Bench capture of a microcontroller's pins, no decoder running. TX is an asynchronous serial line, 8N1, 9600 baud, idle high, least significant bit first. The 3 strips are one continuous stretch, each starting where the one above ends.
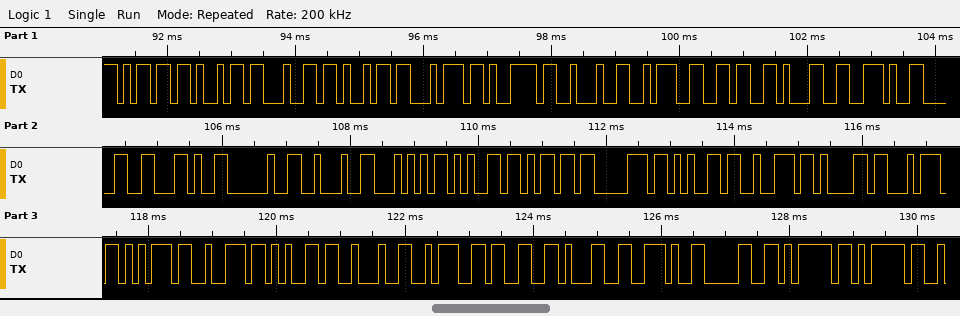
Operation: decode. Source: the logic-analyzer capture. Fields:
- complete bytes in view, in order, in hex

0x6D 0x69 0x64 0x69 0x74 0x79 0x22 0x3A 0x36 0x31 0x2E 0x30 0x2C 0x20 0x22 0x54 0x65 0x6D 0x70 0x65 0x72 0x61 0x74 0x75 0x72 0x65 0x22 0x3A 0x33 0x31 0x2E 0x30 0x7D 0x7D
